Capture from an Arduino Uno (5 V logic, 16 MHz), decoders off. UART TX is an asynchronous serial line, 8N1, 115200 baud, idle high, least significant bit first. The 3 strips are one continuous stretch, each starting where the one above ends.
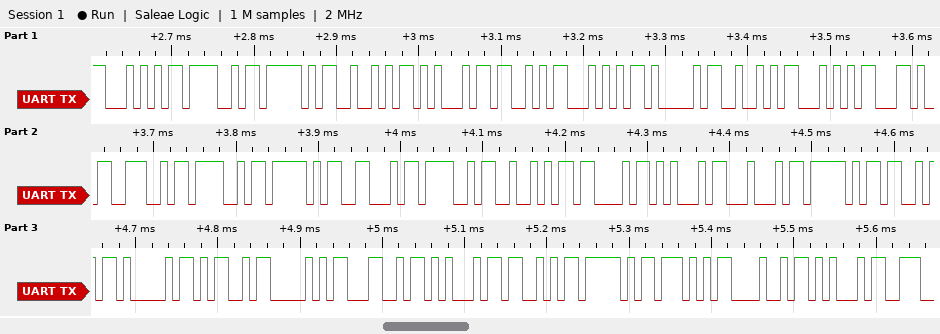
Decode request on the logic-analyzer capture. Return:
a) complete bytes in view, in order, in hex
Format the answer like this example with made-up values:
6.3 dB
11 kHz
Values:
54 4F 5F 52 45 53 54 41 52 54 2C 4E 4F 5F 46 4F 52 43 45 44 5F 53 41 4D 50 4C 45 53 5F 57 48 45
